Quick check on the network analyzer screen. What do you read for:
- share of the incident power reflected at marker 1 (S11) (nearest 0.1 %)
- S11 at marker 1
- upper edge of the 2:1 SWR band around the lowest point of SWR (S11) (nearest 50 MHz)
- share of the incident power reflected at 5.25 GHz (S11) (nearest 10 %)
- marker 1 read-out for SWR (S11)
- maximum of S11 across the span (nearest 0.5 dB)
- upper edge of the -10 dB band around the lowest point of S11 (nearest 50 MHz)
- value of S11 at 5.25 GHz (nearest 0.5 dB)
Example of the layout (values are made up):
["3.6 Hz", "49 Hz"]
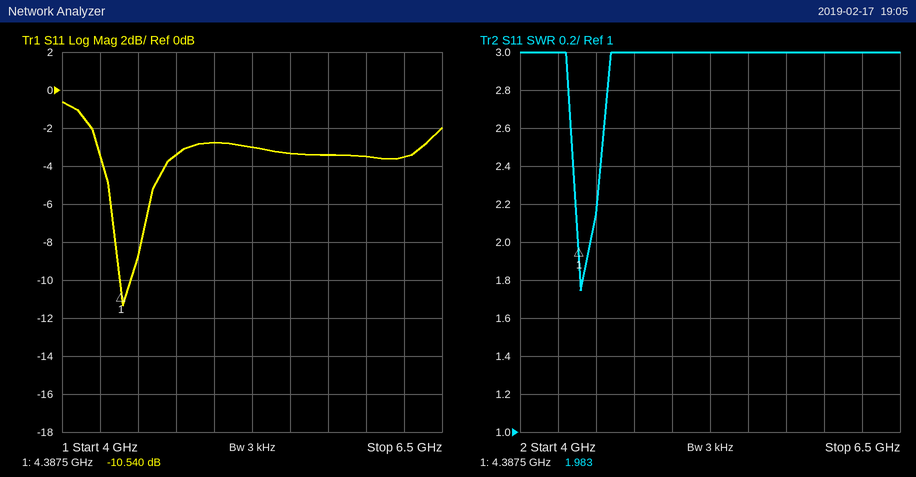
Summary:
["8.8 %", "-10.540 dB", "4.45 GHz", "50 %", "1.983", "-0.5 dB", "4.45 GHz", "-3.0 dB"]
